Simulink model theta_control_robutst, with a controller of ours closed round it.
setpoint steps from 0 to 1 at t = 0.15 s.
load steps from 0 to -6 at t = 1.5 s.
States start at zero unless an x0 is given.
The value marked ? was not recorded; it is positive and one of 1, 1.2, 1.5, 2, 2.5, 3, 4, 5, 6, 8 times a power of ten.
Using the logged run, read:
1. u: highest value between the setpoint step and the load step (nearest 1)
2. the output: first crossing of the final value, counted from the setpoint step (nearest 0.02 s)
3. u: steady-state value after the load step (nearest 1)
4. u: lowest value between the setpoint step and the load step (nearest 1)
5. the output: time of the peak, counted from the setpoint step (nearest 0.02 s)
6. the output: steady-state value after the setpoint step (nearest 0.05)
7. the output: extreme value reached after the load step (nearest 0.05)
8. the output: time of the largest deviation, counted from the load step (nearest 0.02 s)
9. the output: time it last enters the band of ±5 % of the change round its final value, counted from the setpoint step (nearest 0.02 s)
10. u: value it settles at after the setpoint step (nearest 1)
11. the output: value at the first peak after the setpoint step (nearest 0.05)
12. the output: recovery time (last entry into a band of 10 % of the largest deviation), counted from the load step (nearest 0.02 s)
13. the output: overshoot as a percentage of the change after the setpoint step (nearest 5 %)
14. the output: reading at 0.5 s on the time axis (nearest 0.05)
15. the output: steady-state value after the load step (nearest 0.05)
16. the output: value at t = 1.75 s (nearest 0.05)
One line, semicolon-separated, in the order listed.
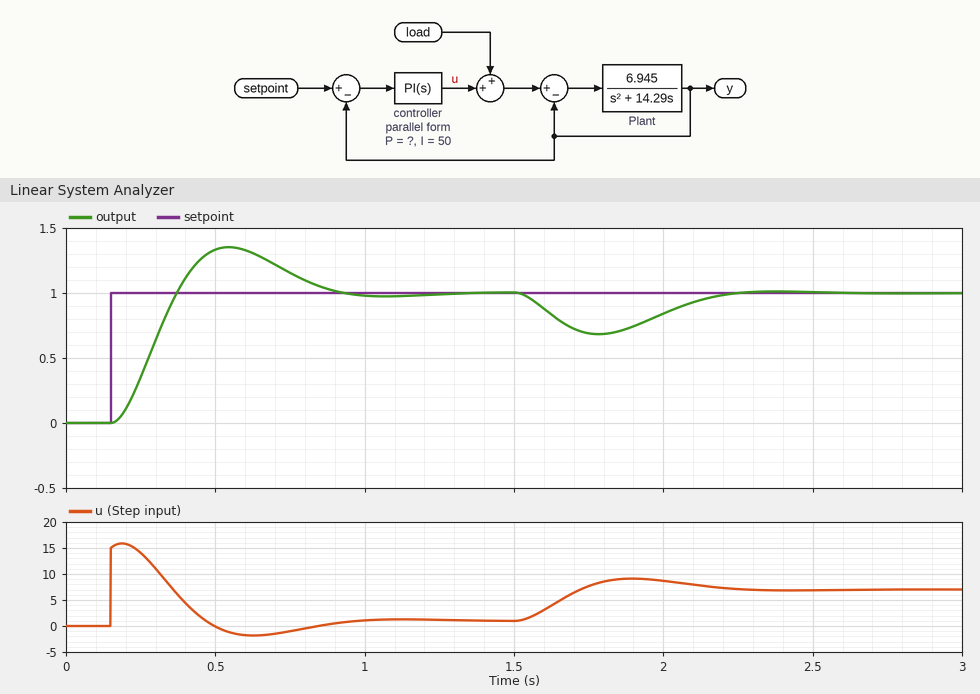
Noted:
16; 0.22 s; 7; -2; 0.40 s; 1.00; 0.70; 0.28 s; 0.70 s; 1; 1.35; 0.66 s; 35 %; 1.35; 1.00; 0.70
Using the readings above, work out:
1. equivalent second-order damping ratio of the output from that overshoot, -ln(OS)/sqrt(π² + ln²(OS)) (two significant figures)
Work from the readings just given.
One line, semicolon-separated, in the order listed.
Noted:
0.32
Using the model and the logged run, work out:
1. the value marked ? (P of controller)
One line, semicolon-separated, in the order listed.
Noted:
15
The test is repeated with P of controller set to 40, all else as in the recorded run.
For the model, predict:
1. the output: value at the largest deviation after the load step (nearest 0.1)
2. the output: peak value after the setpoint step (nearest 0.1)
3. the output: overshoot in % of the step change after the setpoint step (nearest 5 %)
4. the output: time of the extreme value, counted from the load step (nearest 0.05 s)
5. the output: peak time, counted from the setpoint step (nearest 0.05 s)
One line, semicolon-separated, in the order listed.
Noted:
0.8; 1.3; 30 %; 0.20 s; 0.20 s
